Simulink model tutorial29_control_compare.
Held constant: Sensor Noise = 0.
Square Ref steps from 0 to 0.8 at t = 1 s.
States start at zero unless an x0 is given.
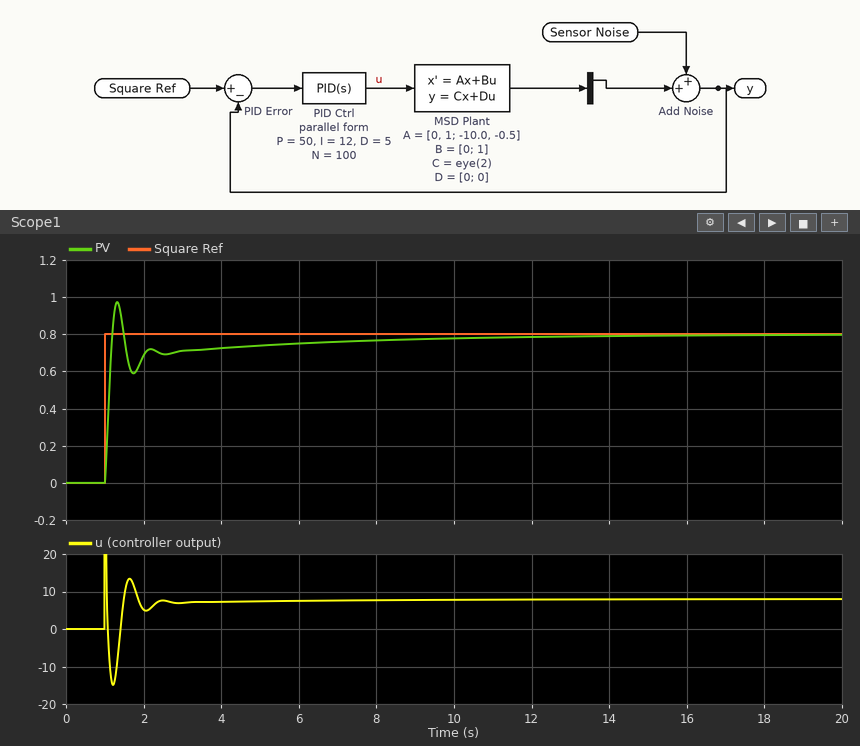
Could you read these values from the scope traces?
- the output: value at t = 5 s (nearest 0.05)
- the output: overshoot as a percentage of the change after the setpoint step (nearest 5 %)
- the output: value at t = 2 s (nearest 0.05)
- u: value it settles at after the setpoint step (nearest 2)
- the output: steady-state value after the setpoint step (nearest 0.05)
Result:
0.75
20 %
0.70
8
0.80
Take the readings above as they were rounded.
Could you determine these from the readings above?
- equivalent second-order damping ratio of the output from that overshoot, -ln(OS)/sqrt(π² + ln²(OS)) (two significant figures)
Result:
0.46
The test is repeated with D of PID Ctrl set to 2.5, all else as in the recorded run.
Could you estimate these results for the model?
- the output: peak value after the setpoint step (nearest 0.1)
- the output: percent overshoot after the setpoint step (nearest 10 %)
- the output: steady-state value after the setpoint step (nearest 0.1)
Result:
1.1
40 %
0.8
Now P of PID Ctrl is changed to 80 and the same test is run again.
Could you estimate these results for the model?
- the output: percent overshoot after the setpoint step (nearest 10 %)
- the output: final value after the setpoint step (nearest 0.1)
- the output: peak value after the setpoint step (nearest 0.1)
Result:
30 %
0.8
1.1
